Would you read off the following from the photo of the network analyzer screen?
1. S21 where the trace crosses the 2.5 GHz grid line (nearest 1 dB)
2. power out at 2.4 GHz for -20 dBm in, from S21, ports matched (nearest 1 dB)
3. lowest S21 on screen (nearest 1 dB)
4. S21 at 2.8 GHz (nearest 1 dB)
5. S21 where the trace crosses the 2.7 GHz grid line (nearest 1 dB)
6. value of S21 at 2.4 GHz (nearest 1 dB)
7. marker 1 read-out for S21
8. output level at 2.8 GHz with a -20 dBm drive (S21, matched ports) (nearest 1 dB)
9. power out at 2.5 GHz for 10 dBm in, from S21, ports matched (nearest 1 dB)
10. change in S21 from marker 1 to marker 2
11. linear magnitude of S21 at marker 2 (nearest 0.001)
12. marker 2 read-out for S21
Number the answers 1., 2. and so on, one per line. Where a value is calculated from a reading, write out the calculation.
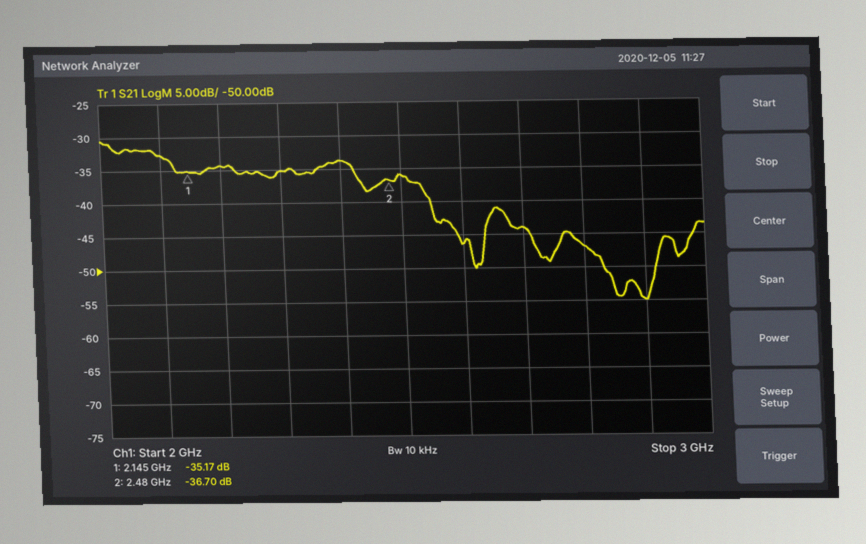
1. -36 dB
2. -20 dBm + (-34 dB) = -54 dBm
3. -55 dB
4. -47 dB
5. -44 dB
6. -34 dB
7. -35.17 dB
8. -20 dBm + (-47 dB) = -67 dBm
9. 10 dBm + (-36 dB) = -26 dBm
10. -36.7 − (-35.17) = -1.53 dB
11. 10^(-36.7/20) ≈ 0.015
12. -36.70 dB
